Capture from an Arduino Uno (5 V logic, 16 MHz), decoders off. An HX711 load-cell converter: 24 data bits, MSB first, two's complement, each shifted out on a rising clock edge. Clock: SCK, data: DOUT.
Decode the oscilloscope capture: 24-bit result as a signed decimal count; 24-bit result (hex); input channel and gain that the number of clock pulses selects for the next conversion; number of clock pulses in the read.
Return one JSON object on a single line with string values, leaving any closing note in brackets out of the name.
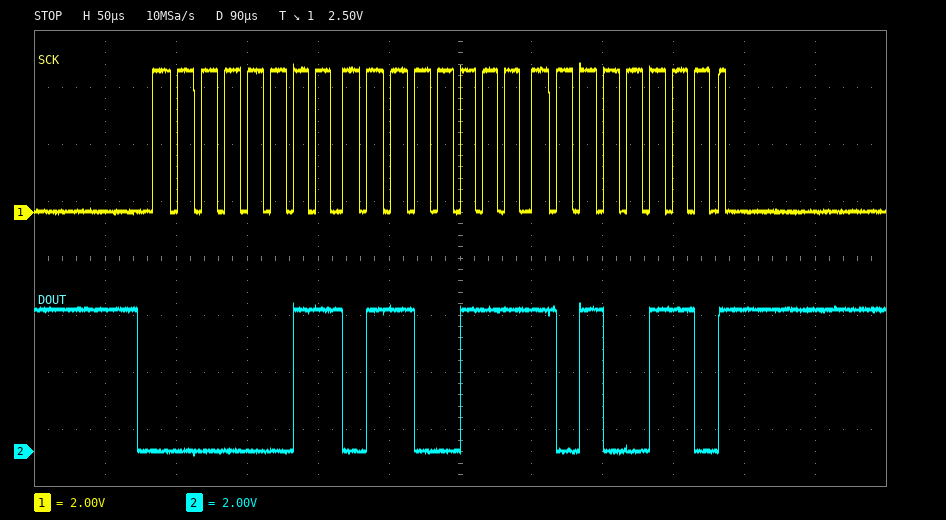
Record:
{"24-bit result as a signed decimal count": "223142", "24-bit result": "0x0367A6", "input channel and gain that the number of clock pulses selects for the next conversion": "channel A, gain 128", "number of clock pulses in the read": "25"}
